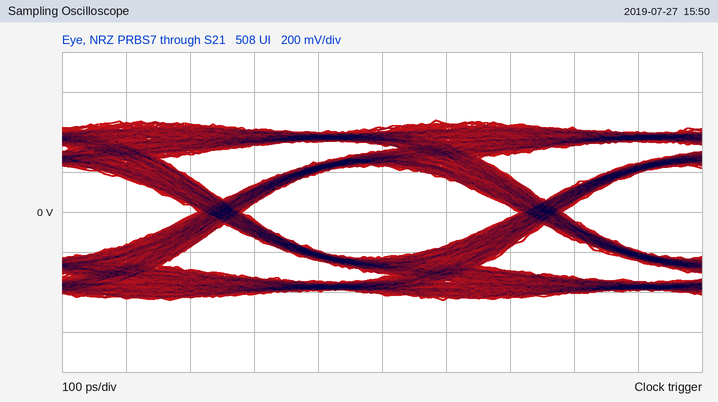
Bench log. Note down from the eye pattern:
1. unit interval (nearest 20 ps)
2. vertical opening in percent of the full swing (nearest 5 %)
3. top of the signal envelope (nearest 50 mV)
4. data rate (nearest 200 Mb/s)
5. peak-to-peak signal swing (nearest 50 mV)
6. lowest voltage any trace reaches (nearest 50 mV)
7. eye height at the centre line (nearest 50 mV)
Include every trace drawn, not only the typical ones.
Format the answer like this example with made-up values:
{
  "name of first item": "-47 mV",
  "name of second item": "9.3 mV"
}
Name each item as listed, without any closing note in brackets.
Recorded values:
{
  "unit interval": "500 ps",
  "vertical opening in percent of the full swing": "50 %",
  "top of the signal envelope": "450 mV",
  "data rate": "2.0 Gb/s",
  "peak-to-peak signal swing": "900 mV",
  "lowest voltage any trace reaches": "-450 mV",
  "eye height at the centre line": "450 mV"
}
